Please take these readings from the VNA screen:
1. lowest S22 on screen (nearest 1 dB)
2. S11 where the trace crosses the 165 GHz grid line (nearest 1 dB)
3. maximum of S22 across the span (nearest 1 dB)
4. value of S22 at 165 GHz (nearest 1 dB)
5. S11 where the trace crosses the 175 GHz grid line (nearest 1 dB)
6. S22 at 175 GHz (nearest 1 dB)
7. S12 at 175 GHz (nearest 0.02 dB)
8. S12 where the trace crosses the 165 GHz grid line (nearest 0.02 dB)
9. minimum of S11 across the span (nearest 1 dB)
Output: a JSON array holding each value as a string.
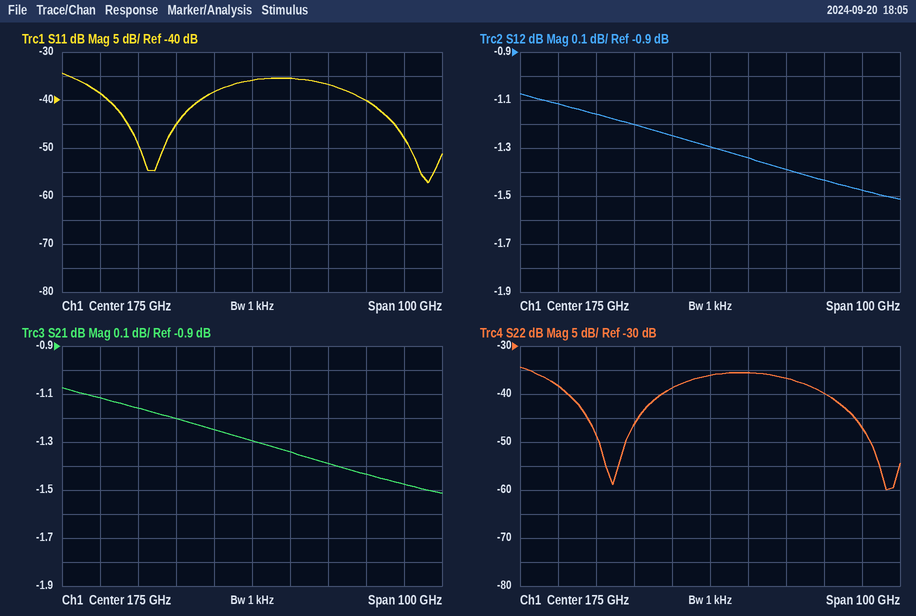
["-60 dB", "-38 dB", "-34 dB", "-39 dB", "-36 dB", "-36 dB", "-1.30 dB", "-1.24 dB", "-57 dB"]
